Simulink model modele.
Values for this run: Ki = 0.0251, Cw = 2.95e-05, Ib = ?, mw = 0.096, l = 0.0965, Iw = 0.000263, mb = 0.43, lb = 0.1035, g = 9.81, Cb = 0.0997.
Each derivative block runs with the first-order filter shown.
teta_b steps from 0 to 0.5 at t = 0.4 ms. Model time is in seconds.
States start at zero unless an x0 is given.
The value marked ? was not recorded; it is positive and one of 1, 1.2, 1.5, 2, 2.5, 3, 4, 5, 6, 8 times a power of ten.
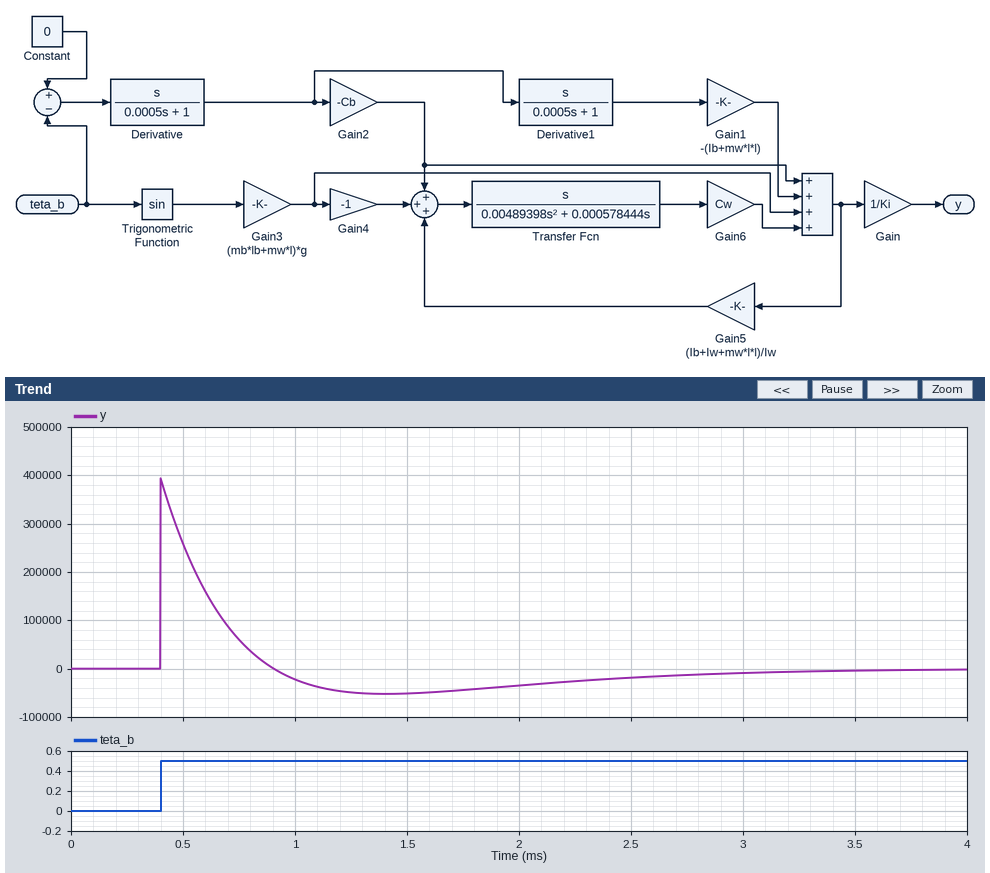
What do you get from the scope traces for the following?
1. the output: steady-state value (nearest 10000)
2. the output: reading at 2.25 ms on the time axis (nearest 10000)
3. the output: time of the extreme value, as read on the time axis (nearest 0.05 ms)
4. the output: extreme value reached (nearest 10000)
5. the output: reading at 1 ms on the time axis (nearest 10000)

0
-30000
0.40 ms
390000
-20000
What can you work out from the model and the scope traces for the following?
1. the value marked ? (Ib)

0.004
